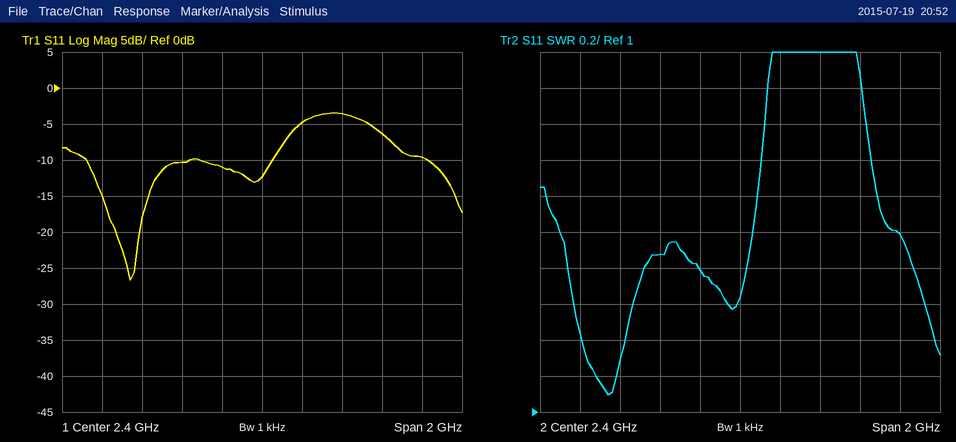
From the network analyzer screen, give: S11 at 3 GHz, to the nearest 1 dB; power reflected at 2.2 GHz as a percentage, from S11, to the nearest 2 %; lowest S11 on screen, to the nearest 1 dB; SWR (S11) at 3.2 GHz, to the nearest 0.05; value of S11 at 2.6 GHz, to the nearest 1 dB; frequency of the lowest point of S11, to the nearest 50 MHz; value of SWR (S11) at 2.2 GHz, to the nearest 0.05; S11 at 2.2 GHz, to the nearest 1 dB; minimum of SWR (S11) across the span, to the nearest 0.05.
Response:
-6 dB
8 %
-27 dB
2.00
-5 dB
1.75 GHz
1.80
-11 dB
1.10
